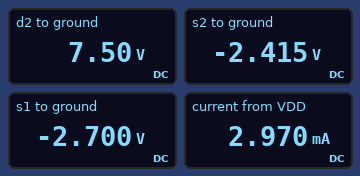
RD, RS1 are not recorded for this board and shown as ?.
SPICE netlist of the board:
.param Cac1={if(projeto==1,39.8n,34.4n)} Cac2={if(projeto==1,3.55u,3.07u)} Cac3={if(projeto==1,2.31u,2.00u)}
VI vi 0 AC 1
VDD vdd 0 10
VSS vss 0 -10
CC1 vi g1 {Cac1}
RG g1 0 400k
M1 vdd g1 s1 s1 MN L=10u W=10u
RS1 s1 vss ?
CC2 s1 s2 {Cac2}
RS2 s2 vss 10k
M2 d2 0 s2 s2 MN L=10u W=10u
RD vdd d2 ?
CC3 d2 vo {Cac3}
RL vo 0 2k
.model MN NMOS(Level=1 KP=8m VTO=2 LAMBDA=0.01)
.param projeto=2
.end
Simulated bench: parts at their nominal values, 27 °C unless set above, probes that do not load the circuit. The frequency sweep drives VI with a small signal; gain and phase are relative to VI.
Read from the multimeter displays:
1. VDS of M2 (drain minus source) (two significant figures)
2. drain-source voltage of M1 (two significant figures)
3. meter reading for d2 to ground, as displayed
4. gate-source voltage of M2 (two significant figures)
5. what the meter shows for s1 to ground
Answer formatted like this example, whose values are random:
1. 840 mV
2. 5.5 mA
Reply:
1. 9.9 V
2. 13 V
3. 7.50 V
4. 2.4 V
5. -2.700 V
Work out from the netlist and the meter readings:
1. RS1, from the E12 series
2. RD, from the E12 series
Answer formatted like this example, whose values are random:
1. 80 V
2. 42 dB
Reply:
1. 3.3 kΩ
2. 3.3 kΩ
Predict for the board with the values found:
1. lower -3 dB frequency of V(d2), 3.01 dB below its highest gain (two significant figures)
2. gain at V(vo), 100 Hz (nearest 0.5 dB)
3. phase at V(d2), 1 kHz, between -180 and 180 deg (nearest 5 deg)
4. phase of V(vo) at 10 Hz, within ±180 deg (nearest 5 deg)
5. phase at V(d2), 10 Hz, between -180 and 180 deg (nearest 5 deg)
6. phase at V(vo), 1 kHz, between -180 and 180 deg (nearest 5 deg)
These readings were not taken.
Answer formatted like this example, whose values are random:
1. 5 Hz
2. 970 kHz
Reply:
1. 110 Hz
2. 4.5 dB
3. 5 deg
4. -170 deg
5. 115 deg
6. 10 deg
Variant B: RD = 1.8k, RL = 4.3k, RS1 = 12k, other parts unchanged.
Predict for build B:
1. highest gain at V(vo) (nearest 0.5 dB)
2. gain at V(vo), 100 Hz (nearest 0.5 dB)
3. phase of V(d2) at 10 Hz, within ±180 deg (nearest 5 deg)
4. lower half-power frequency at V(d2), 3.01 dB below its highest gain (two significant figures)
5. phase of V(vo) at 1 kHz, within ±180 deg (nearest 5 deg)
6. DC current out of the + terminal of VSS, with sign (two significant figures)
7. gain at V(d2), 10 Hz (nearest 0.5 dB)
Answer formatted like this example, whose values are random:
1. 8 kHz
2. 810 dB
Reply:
1. 6.5 dB
2. 4.0 dB
3. 125 deg
4. 93 Hz
5. 5 deg
6. -1.4 mA
7. -14.5 dB
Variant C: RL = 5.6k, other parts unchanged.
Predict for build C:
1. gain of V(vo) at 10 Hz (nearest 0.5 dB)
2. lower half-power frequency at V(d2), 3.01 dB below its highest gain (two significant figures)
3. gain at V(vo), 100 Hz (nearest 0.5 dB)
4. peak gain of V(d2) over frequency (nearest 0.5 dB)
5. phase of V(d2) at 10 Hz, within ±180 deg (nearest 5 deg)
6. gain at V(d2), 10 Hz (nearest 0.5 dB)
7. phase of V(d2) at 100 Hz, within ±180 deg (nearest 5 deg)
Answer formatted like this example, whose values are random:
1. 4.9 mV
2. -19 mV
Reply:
1. -15.0 dB
2. 120 Hz
3. 9.0 dB
4. 13.0 dB
5. 120 deg
6. -10.0 dB
7. 55 deg
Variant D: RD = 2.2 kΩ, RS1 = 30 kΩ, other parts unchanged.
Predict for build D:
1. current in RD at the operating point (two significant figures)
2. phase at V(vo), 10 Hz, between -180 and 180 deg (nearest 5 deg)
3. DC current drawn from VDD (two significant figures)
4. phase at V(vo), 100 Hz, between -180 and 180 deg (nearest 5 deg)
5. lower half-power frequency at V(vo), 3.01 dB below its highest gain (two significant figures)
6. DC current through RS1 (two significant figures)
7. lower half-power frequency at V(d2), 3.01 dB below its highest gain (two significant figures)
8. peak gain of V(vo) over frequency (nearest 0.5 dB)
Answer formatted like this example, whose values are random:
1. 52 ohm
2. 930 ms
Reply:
1. 760 µA
2. -165 deg
3. 1.0 mA
4. 55 deg
5. 78 Hz
6. 260 µA
7. 57 Hz
8. 3.0 dB
